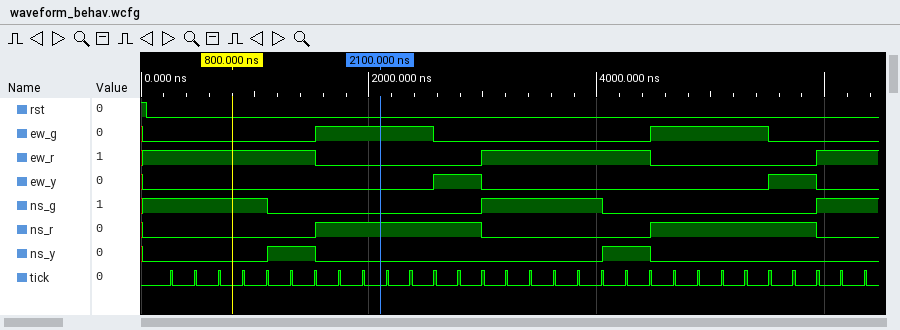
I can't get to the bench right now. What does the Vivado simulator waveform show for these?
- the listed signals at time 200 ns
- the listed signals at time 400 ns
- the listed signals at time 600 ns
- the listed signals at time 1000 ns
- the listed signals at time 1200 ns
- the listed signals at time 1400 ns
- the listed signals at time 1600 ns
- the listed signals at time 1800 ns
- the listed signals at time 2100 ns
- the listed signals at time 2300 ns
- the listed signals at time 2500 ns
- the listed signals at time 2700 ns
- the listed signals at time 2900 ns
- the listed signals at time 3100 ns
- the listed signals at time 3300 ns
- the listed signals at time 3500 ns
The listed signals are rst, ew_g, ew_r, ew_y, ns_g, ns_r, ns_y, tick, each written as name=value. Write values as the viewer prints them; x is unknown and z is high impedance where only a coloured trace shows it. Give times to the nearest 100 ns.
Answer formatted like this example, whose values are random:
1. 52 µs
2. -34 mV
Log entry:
1. rst=0, ew_g=0, ew_r=1, ew_y=0, ns_g=1, ns_r=0, ns_y=0, tick=0
2. rst=0, ew_g=0, ew_r=1, ew_y=0, ns_g=1, ns_r=0, ns_y=0, tick=0
3. rst=0, ew_g=0, ew_r=1, ew_y=0, ns_g=1, ns_r=0, ns_y=0, tick=0
4. rst=0, ew_g=0, ew_r=1, ew_y=0, ns_g=1, ns_r=0, ns_y=0, tick=0
5. rst=0, ew_g=0, ew_r=1, ew_y=0, ns_g=0, ns_r=0, ns_y=1, tick=0
6. rst=0, ew_g=0, ew_r=1, ew_y=0, ns_g=0, ns_r=0, ns_y=1, tick=0
7. rst=0, ew_g=1, ew_r=0, ew_y=0, ns_g=0, ns_r=1, ns_y=0, tick=0
8. rst=0, ew_g=1, ew_r=0, ew_y=0, ns_g=0, ns_r=1, ns_y=0, tick=0
9. rst=0, ew_g=1, ew_r=0, ew_y=0, ns_g=0, ns_r=1, ns_y=0, tick=0
10. rst=0, ew_g=1, ew_r=0, ew_y=0, ns_g=0, ns_r=1, ns_y=0, tick=0
11. rst=0, ew_g=1, ew_r=0, ew_y=0, ns_g=0, ns_r=1, ns_y=0, tick=0
12. rst=0, ew_g=0, ew_r=0, ew_y=1, ns_g=0, ns_r=1, ns_y=0, tick=0
13. rst=0, ew_g=0, ew_r=0, ew_y=1, ns_g=0, ns_r=1, ns_y=0, tick=0
14. rst=0, ew_g=0, ew_r=1, ew_y=0, ns_g=1, ns_r=0, ns_y=0, tick=0
15. rst=0, ew_g=0, ew_r=1, ew_y=0, ns_g=1, ns_r=0, ns_y=0, tick=0
16. rst=0, ew_g=0, ew_r=1, ew_y=0, ns_g=1, ns_r=0, ns_y=0, tick=0
